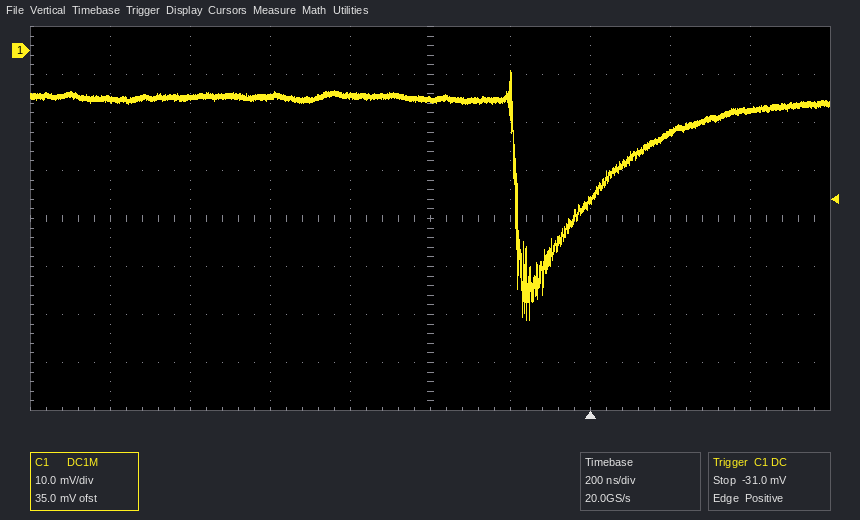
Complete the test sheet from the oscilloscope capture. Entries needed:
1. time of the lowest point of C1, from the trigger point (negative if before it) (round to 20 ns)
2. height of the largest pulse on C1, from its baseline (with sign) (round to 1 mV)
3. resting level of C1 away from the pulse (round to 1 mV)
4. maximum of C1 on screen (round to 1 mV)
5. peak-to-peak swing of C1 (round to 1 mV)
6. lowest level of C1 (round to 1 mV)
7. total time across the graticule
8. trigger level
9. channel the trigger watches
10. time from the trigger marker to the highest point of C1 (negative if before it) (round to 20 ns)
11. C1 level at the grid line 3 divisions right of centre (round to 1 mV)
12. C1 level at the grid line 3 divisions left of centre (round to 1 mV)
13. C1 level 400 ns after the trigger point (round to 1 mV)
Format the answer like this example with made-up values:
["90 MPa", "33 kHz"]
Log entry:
["-160 ns", "-46 mV", "-10 mV", "-4 mV", "52 mV", "-56 mV", "2 µs", "-31.0 mV", "C1", "-200 ns", "-17 mV", "-10 mV", "-12 mV"]
